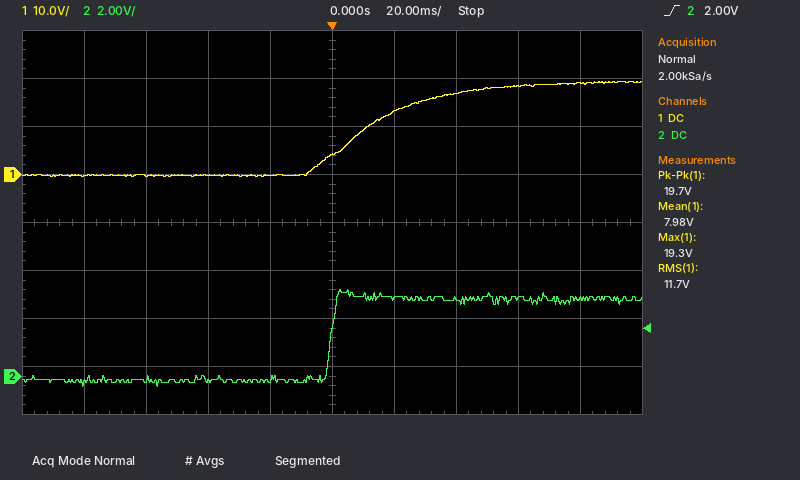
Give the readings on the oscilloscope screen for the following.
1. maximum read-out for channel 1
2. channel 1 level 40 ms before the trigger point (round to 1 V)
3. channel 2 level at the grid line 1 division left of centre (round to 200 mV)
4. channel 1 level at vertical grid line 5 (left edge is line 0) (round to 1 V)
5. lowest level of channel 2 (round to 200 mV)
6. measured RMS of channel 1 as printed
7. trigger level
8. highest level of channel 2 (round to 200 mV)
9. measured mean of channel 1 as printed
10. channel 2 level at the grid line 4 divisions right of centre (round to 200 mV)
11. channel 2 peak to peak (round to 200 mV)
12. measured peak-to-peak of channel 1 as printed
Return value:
19.3 V
0 V
-200 mV
4 V
-400 mV
11.7 V
2.00 V
3.6 V
7.98 V
3.2 V
4.0 V
19.7 V
